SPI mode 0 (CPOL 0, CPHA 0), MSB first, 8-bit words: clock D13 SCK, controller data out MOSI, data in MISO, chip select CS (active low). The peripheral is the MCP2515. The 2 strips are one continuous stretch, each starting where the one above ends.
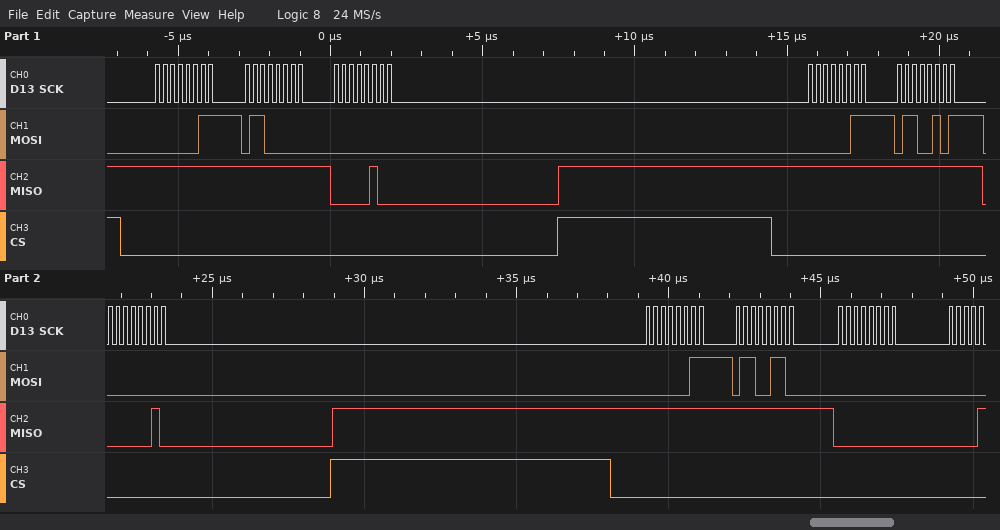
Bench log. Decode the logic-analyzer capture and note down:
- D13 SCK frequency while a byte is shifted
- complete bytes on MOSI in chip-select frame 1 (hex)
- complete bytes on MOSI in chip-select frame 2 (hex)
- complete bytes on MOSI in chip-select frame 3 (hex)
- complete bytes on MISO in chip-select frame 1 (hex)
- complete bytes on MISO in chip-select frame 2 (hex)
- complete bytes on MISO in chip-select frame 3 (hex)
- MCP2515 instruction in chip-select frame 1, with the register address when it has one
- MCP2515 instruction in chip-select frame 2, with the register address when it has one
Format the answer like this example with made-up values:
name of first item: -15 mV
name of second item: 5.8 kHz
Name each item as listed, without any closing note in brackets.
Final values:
D13 SCK frequency while a byte is shifted: 4 MHz
complete bytes on MOSI in chip-select frame 1: 03 60 00
complete bytes on MOSI in chip-select frame 2: 03 65 00
complete bytes on MOSI in chip-select frame 3: 03 66 00
complete bytes on MISO in chip-select frame 1: FF FF 04
complete bytes on MISO in chip-select frame 2: FF FF 02
complete bytes on MISO in chip-select frame 3: FF FF 00
MCP2515 instruction in chip-select frame 1, with the register address when it has one: READ 0x60
MCP2515 instruction in chip-select frame 2, with the register address when it has one: READ 0x65
